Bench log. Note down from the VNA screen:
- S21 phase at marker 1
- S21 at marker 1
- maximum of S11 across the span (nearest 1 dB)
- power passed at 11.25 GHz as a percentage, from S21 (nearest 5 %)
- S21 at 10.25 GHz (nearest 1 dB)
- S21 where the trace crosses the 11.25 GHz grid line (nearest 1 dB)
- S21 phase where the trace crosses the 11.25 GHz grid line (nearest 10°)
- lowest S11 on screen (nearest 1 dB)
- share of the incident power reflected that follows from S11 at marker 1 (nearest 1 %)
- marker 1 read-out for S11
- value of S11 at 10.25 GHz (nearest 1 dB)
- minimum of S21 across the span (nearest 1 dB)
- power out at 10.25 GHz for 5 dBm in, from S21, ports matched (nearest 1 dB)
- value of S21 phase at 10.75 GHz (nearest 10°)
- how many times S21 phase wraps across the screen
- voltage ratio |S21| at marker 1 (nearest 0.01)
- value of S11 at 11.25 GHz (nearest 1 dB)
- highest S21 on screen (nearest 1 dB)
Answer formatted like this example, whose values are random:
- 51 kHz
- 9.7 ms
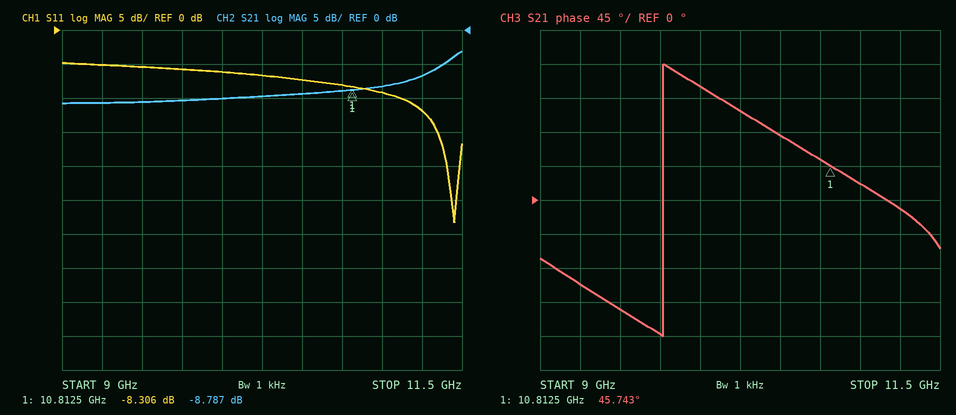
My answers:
- 45.743°
- -8.787 dB
- -5 dB
- 20 %
- -10 dB
- -7 dB
- -10°
- -28 dB
- 15 %
- -8.306 dB
- -7 dB
- -11 dB
- -5 dBm
- 50°
- 1
- 0.36
- -12 dB
- -3 dB
